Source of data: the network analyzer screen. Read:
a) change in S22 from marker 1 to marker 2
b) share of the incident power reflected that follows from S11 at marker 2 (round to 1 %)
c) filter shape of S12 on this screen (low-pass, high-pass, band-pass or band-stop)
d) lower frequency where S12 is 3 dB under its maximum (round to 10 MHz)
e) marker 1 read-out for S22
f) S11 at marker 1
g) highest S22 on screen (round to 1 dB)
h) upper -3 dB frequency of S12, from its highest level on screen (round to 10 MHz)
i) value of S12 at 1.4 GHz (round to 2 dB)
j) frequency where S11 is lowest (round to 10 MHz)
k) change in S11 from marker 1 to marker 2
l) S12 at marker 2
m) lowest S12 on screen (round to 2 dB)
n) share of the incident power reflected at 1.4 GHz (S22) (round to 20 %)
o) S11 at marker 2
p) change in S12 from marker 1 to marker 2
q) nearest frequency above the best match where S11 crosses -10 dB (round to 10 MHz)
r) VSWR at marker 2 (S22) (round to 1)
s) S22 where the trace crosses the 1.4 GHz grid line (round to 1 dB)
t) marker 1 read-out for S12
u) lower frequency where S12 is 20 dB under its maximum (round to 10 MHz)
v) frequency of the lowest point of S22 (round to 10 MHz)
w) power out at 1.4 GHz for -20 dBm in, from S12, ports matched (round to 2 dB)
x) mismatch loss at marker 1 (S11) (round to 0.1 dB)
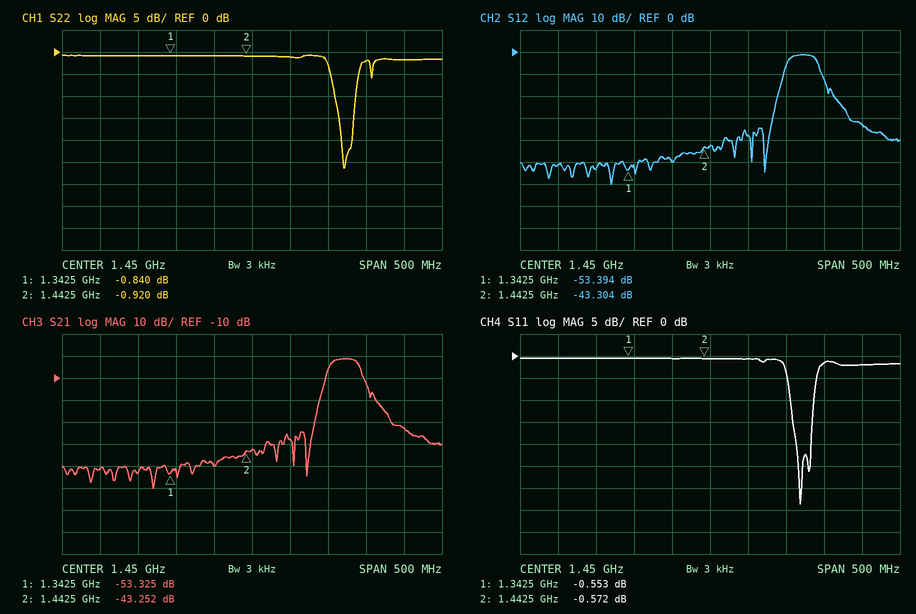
-0.080 dB
88 %
band-pass
1.55 GHz
-0.840 dB
-0.553 dB
-1 dB
1.59 GHz
-50 dB
1.57 GHz
-0.019 dB
-43.304 dB
-60 dB
80 %
-0.572 dB
10.090 dB
1.59 GHz
19
-1 dB
-53.394 dB
1.54 GHz
1.57 GHz
-70 dBm
9.2 dB
